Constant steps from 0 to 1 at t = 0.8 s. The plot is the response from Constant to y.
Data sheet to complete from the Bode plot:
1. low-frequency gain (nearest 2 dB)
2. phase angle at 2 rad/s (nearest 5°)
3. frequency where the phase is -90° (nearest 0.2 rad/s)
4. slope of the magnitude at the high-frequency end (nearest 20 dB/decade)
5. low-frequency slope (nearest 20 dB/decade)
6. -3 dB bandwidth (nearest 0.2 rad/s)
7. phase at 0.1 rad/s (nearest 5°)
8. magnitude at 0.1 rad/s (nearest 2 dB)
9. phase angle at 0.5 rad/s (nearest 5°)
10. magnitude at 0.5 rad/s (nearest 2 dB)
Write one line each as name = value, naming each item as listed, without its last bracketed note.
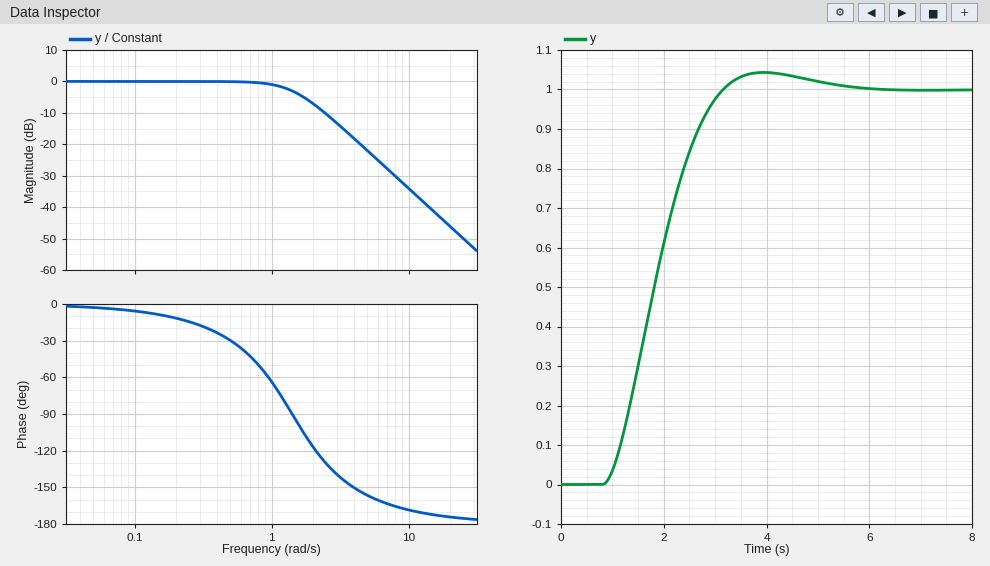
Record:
low-frequency gain = 0 dB
phase angle at 2 rad/s = -115°
frequency where the phase is -90° = 1.4 rad/s
slope of the magnitude at the high-frequency end = -40 dB/decade
low-frequency slope = 0 dB/decade
-3 dB bandwidth = 1.4 rad/s
phase at 0.1 rad/s = -5°
magnitude at 0.1 rad/s = 0 dB
phase angle at 0.5 rad/s = -30°
magnitude at 0.5 rad/s = 0 dB
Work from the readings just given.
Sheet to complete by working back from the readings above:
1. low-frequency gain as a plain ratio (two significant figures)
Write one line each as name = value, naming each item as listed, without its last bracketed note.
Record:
low-frequency gain as a plain ratio = 1.0
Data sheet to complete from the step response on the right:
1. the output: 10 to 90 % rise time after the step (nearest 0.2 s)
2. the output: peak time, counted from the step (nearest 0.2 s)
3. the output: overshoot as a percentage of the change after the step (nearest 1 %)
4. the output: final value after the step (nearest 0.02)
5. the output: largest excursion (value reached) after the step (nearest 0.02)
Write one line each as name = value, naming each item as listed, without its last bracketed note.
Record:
the output: 10 to 90 % rise time after the step = 1.6 s
the output: peak time, counted from the step = 3.2 s
the output: overshoot as a percentage of the change after the step = 4 %
the output: final value after the step = 1.00
the output: largest excursion (value reached) after the step = 1.04
